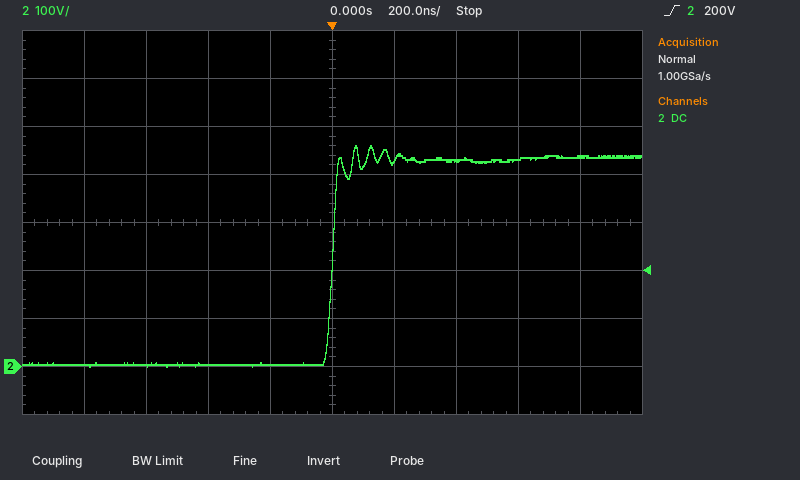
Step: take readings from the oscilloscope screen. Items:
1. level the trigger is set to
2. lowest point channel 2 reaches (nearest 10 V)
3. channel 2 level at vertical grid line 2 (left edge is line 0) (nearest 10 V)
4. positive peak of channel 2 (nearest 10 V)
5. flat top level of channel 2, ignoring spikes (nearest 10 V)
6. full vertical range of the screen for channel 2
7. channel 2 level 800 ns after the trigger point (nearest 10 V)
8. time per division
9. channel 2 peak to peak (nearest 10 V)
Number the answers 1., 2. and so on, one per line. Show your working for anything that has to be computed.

1. 200 V
2. 0 V
3. 0 V
4. 460 V
5. 440 V
6. 800 V
7. 440 V
8. 200 ns
9. 460 V − (0 V) = 460 V
